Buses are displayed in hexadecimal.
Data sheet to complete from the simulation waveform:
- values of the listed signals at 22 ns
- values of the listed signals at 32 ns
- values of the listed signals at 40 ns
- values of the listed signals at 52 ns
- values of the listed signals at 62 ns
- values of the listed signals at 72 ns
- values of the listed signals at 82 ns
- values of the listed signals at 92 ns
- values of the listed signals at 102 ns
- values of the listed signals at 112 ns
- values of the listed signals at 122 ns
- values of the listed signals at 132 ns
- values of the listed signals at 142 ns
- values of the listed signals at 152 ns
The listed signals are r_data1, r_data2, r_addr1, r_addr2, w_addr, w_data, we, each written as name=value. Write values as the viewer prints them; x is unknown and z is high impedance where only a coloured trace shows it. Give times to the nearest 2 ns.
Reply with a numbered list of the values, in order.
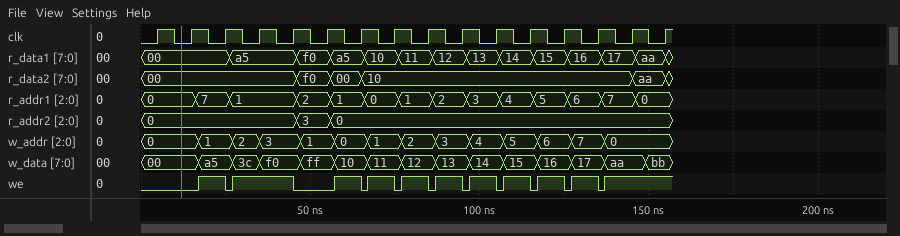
1. r_data1=00, r_data2=00, r_addr1=7, r_addr2=0, w_addr=1, w_data=a5, we=1
2. r_data1=a5, r_data2=00, r_addr1=1, r_addr2=0, w_addr=2, w_data=3c, we=1
3. r_data1=a5, r_data2=00, r_addr1=1, r_addr2=0, w_addr=3, w_data=f0, we=1
4. r_data1=f0, r_data2=f0, r_addr1=2, r_addr2=3, w_addr=1, w_data=ff, we=0
5. r_data1=a5, r_data2=00, r_addr1=1, r_addr2=0, w_addr=0, w_data=10, we=1
6. r_data1=10, r_data2=10, r_addr1=0, r_addr2=0, w_addr=1, w_data=11, we=1
7. r_data1=11, r_data2=10, r_addr1=1, r_addr2=0, w_addr=2, w_data=12, we=1
8. r_data1=12, r_data2=10, r_addr1=2, r_addr2=0, w_addr=3, w_data=13, we=1
9. r_data1=13, r_data2=10, r_addr1=3, r_addr2=0, w_addr=4, w_data=14, we=1
10. r_data1=14, r_data2=10, r_addr1=4, r_addr2=0, w_addr=5, w_data=15, we=1
11. r_data1=15, r_data2=10, r_addr1=5, r_addr2=0, w_addr=6, w_data=16, we=1
12. r_data1=16, r_data2=10, r_addr1=6, r_addr2=0, w_addr=7, w_data=17, we=1
13. r_data1=17, r_data2=10, r_addr1=7, r_addr2=0, w_addr=0, w_data=aa, we=1
14. r_data1=aa, r_data2=aa, r_addr1=0, r_addr2=0, w_addr=0, w_data=bb, we=1
